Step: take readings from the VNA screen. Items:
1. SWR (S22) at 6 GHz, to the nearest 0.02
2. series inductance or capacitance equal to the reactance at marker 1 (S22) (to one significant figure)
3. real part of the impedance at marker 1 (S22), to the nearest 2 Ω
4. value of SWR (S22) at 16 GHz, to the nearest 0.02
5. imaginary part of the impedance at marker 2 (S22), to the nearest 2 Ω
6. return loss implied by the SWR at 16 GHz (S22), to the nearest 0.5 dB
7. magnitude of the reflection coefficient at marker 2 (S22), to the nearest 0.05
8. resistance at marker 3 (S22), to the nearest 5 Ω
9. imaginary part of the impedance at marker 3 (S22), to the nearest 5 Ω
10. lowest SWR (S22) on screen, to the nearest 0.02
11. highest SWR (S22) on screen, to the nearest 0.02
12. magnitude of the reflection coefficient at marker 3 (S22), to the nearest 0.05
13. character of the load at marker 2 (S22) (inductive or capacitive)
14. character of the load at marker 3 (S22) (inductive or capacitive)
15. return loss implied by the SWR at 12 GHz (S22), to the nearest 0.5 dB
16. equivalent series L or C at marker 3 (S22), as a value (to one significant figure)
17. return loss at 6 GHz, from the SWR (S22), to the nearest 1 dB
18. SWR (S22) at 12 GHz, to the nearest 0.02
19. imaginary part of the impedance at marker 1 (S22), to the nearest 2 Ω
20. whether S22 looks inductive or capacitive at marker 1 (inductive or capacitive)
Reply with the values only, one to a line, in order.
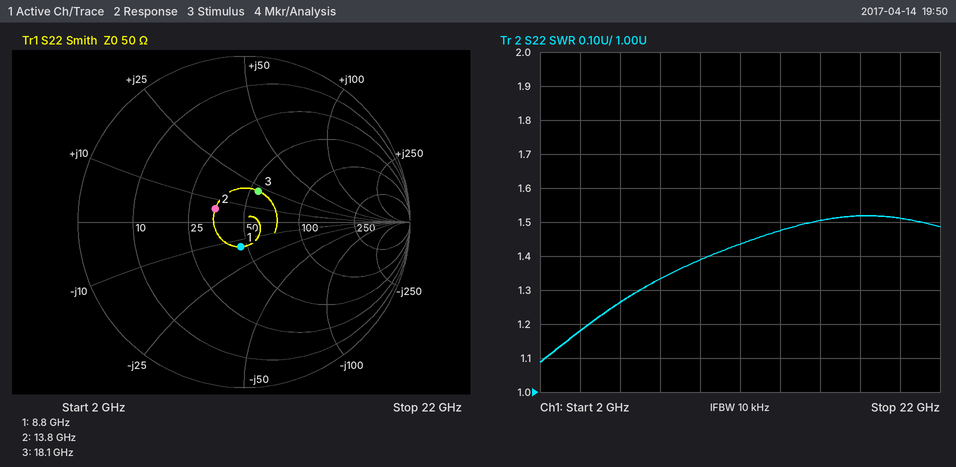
1.26
1 pF
46 Ω
1.50
+6 Ω
14.0 dB
0.20
55 Ω
+20 Ω
1.08
1.52
0.20
inductive
inductive
15.0 dB
200 pH
19 dB
1.44
-14 Ω
capacitive
